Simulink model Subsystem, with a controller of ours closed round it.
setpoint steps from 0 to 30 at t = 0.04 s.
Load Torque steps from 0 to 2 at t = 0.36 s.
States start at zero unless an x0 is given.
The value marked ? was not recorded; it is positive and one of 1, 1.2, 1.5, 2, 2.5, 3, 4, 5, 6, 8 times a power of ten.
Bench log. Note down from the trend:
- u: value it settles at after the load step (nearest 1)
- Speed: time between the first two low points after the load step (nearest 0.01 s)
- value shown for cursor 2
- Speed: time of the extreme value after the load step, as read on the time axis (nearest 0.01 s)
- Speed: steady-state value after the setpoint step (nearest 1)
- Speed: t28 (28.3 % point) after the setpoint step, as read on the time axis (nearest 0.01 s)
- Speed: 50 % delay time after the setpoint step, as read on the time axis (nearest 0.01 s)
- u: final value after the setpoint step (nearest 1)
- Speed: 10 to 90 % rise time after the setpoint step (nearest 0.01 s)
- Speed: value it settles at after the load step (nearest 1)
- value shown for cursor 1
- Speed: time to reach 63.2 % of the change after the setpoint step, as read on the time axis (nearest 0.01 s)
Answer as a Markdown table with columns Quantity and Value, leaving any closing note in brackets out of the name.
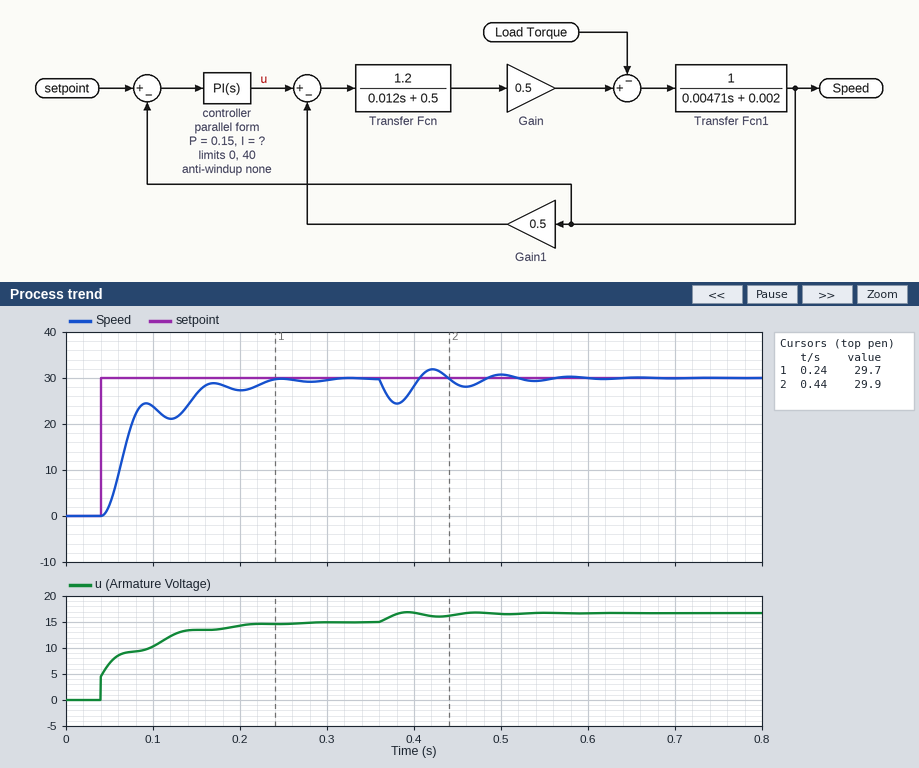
| Quantity | Value |
|---|---|
| u: value it settles at after the load step | 17 |
| Speed: time between the first two low points after the load step | 0.08 s |
| value shown for cursor 2 | 29.9 |
| Speed: time of the extreme value after the load step, as read on the time axis | 0.38 s |
| Speed: steady-state value after the setpoint step | 30 |
| Speed: t28 (28.3 % point) after the setpoint step, as read on the time axis | 0.06 s |
| Speed: 50 % delay time after the setpoint step, as read on the time axis | 0.07 s |
| u: final value after the setpoint step | 15 |
| Speed: 10 to 90 % rise time after the setpoint step | 0.10 s |
| Speed: value it settles at after the load step | 30 |
| value shown for cursor 1 | 29.7 |
| Speed: time to reach 63.2 % of the change after the setpoint step, as read on the time axis | 0.07 s |
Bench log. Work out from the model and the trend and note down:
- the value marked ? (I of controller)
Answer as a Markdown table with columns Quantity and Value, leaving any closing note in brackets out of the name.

| Quantity | Value |
|---|---|
| the value marked ? | 10 |
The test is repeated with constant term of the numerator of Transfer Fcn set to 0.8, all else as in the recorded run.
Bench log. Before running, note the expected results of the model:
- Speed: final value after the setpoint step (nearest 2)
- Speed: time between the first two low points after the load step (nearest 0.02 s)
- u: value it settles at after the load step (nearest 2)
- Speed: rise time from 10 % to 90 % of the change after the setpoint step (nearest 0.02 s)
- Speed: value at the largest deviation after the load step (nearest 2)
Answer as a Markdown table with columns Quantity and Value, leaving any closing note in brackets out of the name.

| Quantity | Value |
|---|---|
| Speed: final value after the setpoint step | 30 |
| Speed: time between the first two low points after the load step | 0.10 s |
| u: value it settles at after the load step | 18 |
| Speed: rise time from 10 % to 90 % of the change after the setpoint step | 0.12 s |
| Speed: value at the largest deviation after the load step | 24 |
